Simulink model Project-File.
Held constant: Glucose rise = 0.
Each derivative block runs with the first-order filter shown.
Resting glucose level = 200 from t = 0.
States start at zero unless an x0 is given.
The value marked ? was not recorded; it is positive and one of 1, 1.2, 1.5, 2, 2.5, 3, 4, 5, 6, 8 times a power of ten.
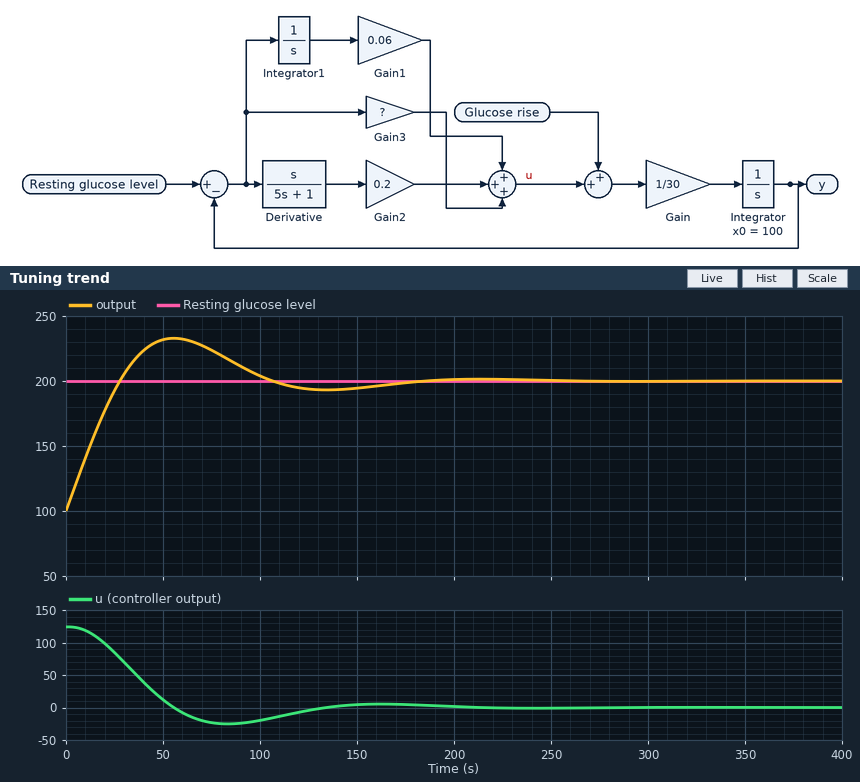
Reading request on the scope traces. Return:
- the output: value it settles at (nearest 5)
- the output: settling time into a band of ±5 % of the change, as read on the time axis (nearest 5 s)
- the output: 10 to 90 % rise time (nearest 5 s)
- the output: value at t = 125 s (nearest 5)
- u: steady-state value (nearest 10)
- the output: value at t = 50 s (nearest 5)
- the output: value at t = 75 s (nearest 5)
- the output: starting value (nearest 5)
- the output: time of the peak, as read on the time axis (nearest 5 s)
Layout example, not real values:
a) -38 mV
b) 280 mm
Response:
a) 200
b) 155 s
c) 20 s
d) 195
e) 0
f) 230
g) 225
h) 100
i) 55 s
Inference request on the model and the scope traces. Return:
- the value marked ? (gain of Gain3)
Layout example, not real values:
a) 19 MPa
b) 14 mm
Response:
a) 1.2
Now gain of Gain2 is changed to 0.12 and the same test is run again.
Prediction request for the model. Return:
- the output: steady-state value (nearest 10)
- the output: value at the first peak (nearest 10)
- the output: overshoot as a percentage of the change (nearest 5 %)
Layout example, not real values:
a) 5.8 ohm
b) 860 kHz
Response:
a) 200
b) 230
c) 35 %
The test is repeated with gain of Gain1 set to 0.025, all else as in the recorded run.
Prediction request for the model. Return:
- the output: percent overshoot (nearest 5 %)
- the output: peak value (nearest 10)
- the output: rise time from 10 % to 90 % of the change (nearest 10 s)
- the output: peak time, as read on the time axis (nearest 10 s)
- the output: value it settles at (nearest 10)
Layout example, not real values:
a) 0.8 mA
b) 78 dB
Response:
a) 20 %
b) 220
c) 30 s
d) 80 s
e) 200
